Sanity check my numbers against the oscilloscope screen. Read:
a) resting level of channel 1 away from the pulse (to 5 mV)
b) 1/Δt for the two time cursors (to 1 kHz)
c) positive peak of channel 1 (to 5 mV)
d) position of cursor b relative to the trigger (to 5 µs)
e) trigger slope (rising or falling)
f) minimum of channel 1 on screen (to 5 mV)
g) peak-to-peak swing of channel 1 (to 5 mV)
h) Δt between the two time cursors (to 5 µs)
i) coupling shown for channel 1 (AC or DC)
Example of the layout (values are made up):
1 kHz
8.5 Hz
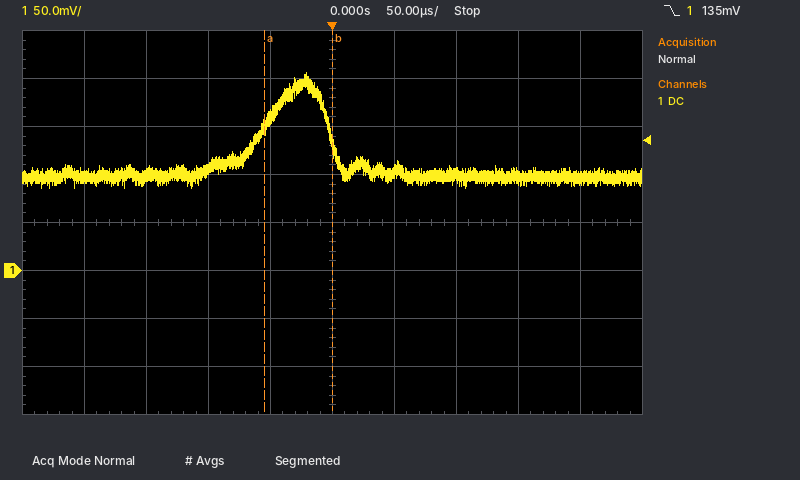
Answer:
100 mV
18 kHz
205 mV
0 µs
falling
85 mV
120 mV
55 µs
DC
